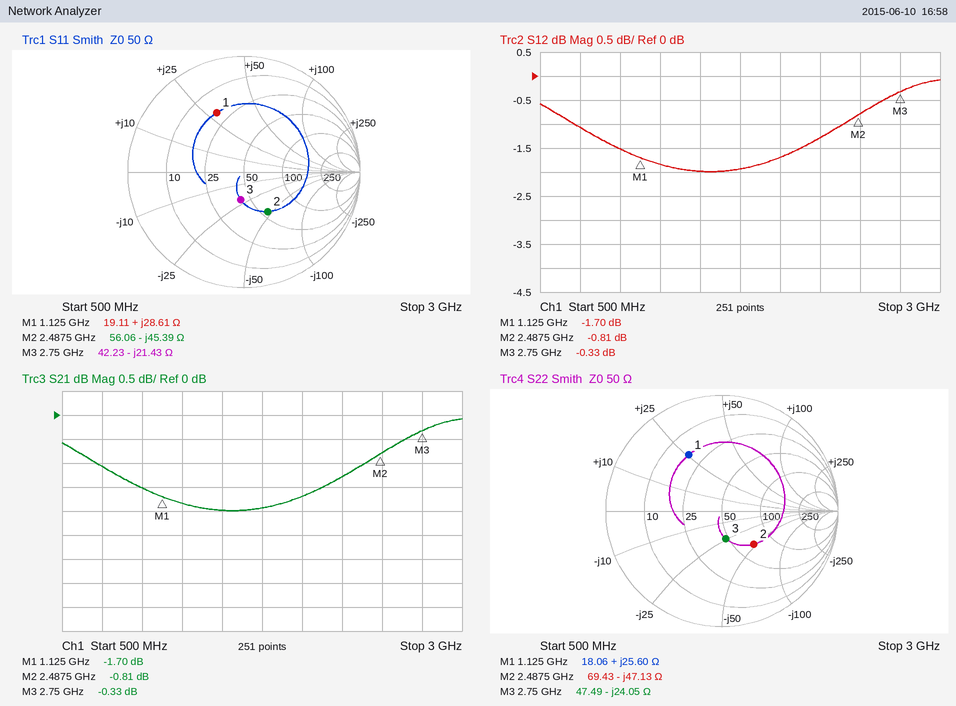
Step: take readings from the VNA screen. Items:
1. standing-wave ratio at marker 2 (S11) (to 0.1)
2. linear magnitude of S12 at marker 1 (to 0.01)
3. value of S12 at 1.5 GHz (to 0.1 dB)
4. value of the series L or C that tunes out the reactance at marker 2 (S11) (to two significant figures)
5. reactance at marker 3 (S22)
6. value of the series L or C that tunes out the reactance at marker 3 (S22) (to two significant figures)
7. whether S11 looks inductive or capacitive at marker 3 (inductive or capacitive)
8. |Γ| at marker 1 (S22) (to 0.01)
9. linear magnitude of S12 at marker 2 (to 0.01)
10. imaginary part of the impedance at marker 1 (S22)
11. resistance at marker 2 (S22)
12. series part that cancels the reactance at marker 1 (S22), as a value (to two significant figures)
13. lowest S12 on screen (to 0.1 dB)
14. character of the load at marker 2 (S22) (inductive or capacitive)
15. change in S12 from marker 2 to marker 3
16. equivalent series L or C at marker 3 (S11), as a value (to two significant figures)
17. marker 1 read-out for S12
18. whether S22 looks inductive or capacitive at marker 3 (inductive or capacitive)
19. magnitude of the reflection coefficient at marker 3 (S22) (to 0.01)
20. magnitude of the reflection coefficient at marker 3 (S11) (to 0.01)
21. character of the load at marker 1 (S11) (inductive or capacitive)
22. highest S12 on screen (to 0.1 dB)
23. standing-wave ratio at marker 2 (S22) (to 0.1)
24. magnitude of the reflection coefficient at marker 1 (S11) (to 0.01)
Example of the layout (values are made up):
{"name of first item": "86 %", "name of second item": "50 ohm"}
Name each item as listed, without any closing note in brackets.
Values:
{"standing-wave ratio at marker 2 (S11)": "2.3", "linear magnitude of S12 at marker 1": "0.82", "value of S12 at 1.5 GHz": "-2.0 dB", "value of the series L or C that tunes out the reactance at marker 2 (S11)": "2.9 nH", "reactance at marker 3": "-24.05 Ω", "value of the series L or C that tunes out the reactance at marker 3 (S22)": "1.4 nH", "whether S11 looks inductive or capacitive at marker 3": "capacitive", "|Γ| at marker 1 (S22)": "0.56", "linear magnitude of S12 at marker 2": "0.91", "imaginary part of the impedance at marker 1": "+25.60 Ω", "resistance at marker 2": "69.43 Ω", "series part that cancels the reactance at marker 1 (S22), as a value": "5.5 pF", "lowest S12 on screen": "-2.0 dB", "character of the load at marker 2 (S22)": "capacitive", "change in S12 from marker 2 to marker 3": "0.48 dB", "equivalent series L or C at marker 3 (S11), as a value": "2.7 pF", "marker 1 read-out for S12": "-1.70 dB", "whether S22 looks inductive or capacitive at marker 3": "capacitive", "magnitude of the reflection coefficient at marker 3 (S22)": "0.24", "magnitude of the reflection coefficient at marker 3 (S11)": "0.24", "character of the load at marker 1 (S11)": "inductive", "highest S12 on screen": "-0.1 dB", "standing-wave ratio at marker 2 (S22)": "2.3", "magnitude of the reflection coefficient at marker 1 (S11)": "0.56"}
